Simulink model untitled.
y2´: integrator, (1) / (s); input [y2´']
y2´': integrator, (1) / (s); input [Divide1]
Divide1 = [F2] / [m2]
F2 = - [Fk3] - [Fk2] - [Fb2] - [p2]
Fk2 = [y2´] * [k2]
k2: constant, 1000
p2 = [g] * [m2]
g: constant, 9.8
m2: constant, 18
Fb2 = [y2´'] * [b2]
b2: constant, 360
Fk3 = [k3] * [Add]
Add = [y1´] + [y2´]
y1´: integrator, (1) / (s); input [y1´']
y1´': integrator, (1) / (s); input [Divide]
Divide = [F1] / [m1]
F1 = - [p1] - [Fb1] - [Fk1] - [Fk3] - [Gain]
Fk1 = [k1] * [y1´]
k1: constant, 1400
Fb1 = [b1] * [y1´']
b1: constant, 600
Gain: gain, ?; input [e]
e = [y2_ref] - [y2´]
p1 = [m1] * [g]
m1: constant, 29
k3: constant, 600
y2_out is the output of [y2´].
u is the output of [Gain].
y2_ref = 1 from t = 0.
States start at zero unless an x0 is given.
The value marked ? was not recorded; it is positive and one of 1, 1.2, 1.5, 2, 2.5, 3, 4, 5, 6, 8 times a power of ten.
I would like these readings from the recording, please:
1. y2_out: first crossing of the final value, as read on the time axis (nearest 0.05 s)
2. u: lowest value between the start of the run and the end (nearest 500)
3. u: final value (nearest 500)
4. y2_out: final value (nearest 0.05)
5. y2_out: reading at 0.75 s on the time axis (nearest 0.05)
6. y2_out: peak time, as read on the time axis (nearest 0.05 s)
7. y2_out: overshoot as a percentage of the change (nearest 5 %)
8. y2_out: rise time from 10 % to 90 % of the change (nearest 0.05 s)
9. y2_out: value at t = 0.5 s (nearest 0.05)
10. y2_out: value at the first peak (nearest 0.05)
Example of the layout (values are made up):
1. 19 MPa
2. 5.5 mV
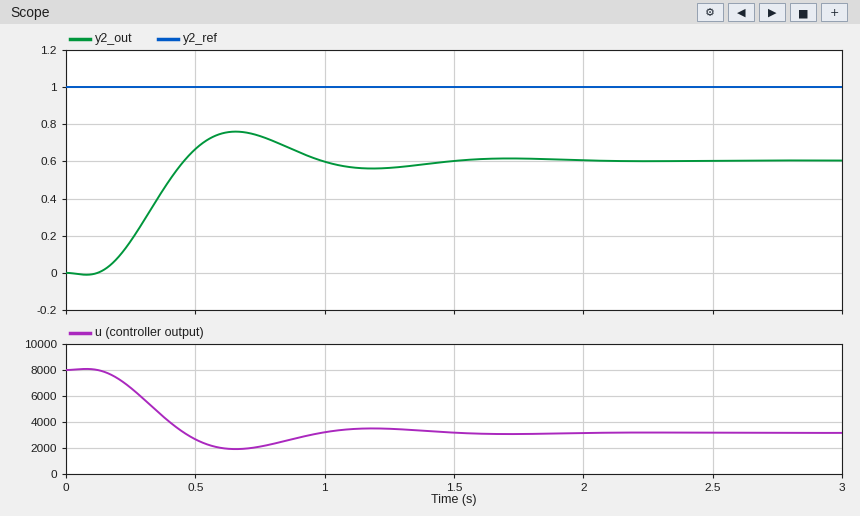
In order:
1. 0.45 s
2. 2000
3. 3000
4. 0.60
5. 0.75
6. 0.65 s
7. 25 %
8. 0.25 s
9. 0.65
10. 0.75
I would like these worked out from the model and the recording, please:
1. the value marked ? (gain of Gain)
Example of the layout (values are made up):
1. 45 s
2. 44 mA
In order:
1. 8000
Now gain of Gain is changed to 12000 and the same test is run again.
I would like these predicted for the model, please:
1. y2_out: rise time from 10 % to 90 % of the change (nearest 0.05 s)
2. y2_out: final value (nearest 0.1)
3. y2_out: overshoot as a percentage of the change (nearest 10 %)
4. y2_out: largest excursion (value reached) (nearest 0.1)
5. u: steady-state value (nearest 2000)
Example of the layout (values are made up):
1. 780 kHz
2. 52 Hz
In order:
1. 0.20 s
2. 0.7
3. 40 %
4. 1.0
5. 4000
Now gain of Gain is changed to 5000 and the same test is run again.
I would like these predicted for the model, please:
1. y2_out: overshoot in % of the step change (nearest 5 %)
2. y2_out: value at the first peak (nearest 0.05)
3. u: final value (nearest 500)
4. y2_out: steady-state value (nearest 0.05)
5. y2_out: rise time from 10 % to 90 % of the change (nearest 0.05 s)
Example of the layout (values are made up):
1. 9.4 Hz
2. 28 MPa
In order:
1. 15 %
2. 0.55
3. 2500
4. 0.50
5. 0.30 s
